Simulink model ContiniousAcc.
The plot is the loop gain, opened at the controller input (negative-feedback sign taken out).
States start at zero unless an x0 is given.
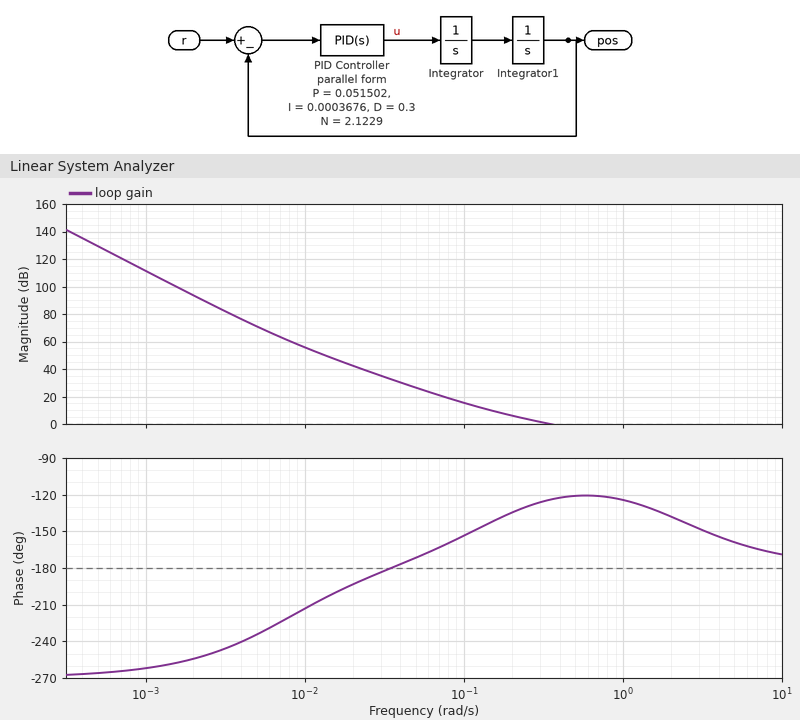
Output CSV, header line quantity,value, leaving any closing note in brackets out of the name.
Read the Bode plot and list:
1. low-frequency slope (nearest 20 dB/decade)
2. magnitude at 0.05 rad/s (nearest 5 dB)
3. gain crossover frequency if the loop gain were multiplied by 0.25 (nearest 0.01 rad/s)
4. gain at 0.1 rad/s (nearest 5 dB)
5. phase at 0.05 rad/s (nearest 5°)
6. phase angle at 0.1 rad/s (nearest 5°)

quantity,value
low-frequency slope,-60 dB/decade
magnitude at 0.05 rad/s,25 dB
gain crossover frequency if the loop gain were multiplied by 0.25,0.13 rad/s
gain at 0.1 rad/s,15 dB
phase at 0.05 rad/s,-170°
phase angle at 0.1 rad/s,-155°
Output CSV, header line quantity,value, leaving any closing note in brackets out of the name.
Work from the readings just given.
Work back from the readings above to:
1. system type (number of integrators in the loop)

quantity,value
system type,3
